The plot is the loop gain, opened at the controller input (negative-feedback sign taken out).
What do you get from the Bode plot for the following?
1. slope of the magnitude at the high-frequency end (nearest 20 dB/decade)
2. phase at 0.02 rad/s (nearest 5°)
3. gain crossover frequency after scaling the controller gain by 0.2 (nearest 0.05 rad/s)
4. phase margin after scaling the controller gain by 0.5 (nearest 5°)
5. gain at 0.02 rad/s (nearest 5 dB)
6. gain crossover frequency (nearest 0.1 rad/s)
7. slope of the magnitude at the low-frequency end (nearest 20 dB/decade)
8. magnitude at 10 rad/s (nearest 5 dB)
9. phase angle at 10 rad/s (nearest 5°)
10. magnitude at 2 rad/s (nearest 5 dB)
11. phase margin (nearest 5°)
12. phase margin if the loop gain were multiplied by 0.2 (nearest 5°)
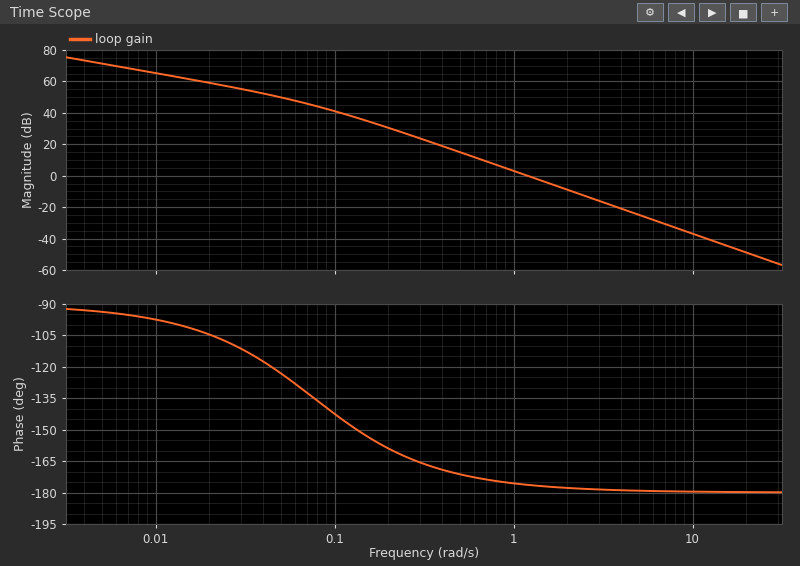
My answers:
-40 dB/decade
-105°
0.55 rad/s
5°
60 dB
1.2 rad/s
-20 dB/decade
-35 dB
-180°
-10 dB
5°
10°
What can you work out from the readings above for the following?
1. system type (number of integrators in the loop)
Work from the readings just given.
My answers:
1
